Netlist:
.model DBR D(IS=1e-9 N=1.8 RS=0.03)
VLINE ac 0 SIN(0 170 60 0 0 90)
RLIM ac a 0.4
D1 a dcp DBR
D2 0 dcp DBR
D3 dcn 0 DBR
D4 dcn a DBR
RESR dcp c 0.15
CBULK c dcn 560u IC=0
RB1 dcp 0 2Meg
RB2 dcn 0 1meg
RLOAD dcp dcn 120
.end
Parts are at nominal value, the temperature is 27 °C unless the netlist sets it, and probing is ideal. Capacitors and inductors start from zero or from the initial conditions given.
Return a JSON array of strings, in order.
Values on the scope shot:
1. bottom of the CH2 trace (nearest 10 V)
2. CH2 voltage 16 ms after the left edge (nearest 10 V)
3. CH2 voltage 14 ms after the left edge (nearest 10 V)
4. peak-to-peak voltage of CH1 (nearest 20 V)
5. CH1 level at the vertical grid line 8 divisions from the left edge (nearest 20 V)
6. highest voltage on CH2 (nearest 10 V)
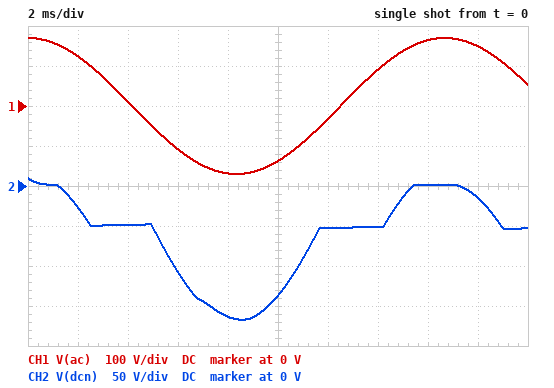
["-170 V", "0 V", "-50 V", "340 V", "160 V", "10 V"]
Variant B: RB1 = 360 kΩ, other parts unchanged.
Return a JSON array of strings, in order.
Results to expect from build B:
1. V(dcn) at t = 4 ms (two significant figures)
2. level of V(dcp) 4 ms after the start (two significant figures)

["-110 V", "39 V"]
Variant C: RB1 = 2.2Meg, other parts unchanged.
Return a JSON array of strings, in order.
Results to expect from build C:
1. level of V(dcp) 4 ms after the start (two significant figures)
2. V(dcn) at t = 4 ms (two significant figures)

["100 V", "-46 V"]
